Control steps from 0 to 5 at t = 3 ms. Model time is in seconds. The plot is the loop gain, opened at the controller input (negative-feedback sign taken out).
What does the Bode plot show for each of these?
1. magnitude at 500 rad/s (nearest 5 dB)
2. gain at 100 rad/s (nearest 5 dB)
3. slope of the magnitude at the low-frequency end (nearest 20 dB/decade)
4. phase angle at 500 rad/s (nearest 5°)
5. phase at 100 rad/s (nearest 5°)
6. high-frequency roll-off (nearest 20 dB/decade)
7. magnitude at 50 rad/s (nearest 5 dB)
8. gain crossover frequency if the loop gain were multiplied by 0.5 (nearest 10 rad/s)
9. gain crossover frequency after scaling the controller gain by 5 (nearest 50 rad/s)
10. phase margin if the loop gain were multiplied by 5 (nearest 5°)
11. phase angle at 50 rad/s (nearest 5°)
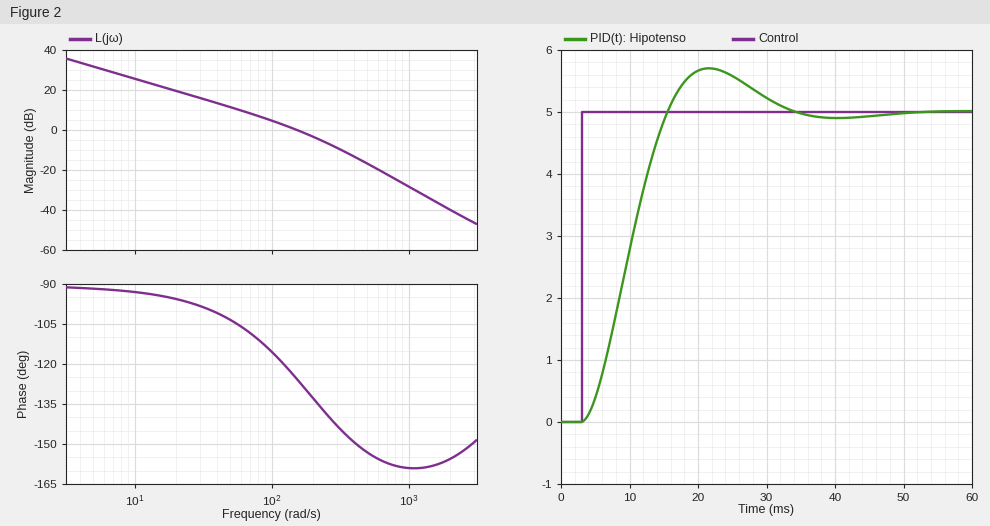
-15 dB
5 dB
-20 dB/decade
-155°
-115°
-40 dB/decade
10 dB
90 rad/s
400 rad/s
30°
-105°
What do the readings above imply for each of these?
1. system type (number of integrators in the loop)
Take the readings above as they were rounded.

1
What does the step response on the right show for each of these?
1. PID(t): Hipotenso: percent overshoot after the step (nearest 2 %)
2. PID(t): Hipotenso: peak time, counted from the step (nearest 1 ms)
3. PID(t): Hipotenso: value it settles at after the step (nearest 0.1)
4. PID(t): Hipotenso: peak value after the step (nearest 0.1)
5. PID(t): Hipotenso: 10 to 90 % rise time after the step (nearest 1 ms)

14 %
19 ms
5.0
5.7
9 ms
